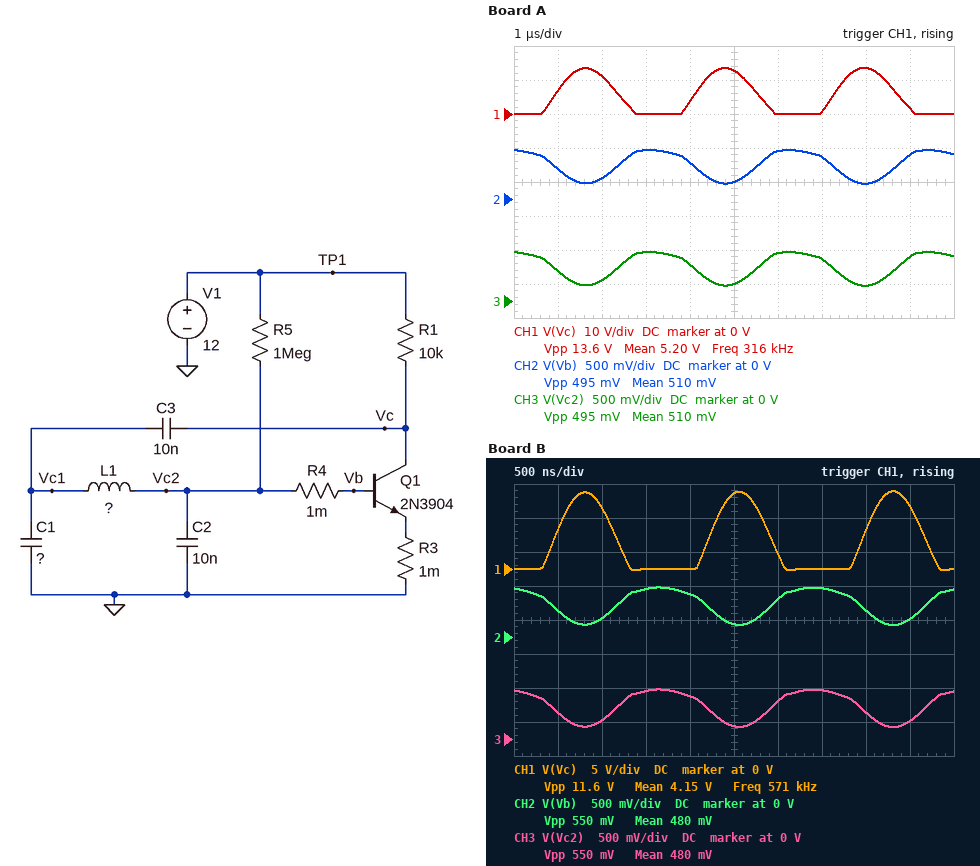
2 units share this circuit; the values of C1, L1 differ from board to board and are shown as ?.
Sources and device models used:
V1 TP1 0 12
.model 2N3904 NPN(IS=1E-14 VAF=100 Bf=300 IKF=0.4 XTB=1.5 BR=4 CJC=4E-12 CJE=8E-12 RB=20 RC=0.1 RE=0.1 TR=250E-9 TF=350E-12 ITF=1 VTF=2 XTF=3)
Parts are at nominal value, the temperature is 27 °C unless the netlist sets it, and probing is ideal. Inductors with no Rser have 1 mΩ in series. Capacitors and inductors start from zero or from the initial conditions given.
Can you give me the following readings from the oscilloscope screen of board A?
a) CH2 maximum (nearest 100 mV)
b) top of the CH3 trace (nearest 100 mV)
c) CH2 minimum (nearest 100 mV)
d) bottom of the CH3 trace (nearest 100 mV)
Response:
700 mV
700 mV
200 mV
200 mV
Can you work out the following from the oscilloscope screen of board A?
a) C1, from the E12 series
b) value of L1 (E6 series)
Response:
330 pF
680 µH
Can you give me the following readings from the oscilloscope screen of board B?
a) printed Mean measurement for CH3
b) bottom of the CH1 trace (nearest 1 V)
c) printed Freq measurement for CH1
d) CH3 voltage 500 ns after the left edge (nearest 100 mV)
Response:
480 mV
0 V
571 kHz
400 mV
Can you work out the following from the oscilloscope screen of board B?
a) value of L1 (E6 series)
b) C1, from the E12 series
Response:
150 µH
390 pF
